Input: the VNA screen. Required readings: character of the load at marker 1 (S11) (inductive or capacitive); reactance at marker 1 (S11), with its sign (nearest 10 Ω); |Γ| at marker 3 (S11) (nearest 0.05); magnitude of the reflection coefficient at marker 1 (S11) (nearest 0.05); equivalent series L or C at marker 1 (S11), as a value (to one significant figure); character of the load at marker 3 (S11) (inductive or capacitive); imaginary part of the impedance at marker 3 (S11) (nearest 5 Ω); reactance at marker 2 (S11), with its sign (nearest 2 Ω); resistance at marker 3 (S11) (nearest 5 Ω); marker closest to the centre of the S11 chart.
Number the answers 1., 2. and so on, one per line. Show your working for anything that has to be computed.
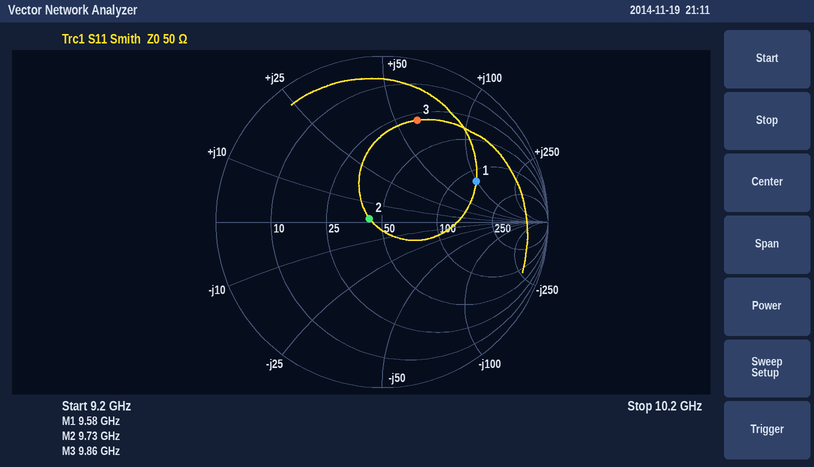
1. inductive
2. +100 Ω
3. 0.65
4. 0.60
5. L = 100 Ω/(2π × 9.58 GHz) ≈ 2 nH
6. inductive
7. +60 Ω
8. +2 Ω
9. 30 Ω
10. marker 2
